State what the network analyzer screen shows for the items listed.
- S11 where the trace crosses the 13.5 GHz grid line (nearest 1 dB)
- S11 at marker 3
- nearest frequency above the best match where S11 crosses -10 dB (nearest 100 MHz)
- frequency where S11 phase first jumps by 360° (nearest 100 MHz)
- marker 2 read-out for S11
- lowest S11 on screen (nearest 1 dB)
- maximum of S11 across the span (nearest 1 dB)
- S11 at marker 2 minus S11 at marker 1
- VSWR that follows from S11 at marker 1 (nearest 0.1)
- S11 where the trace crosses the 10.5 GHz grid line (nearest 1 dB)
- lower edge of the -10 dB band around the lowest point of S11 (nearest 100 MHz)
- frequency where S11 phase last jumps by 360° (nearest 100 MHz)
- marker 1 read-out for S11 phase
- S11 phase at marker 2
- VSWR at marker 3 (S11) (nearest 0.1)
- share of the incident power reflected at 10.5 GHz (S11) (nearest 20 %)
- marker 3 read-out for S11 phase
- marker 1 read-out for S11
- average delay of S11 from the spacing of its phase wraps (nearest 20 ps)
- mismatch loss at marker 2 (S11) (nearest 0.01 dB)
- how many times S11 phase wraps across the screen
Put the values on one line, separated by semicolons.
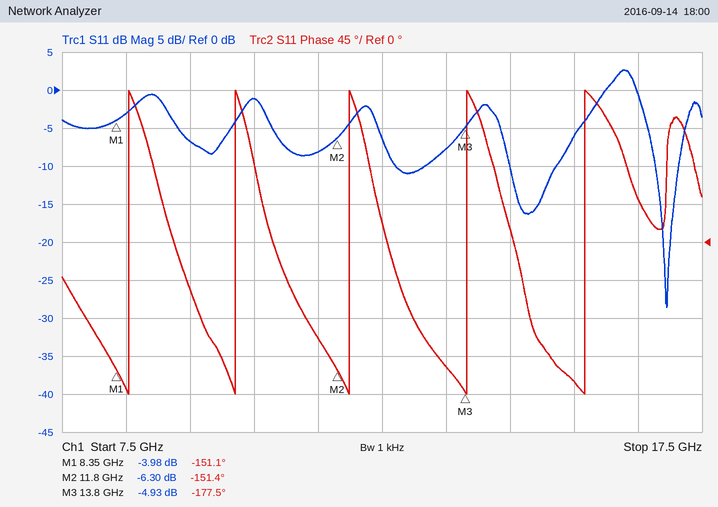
-8 dB; -4.93 dB; 17.1 GHz; 8.5 GHz; -6.30 dB; -29 dB; 3 dB; -2.32 dB; 4.4; -1 dB; 16.8 GHz; 15.7 GHz; -151.1°; -151.4°; 3.6; 80 %; -177.5°; -3.98 dB; 560 ps; 1.16 dB; 5
